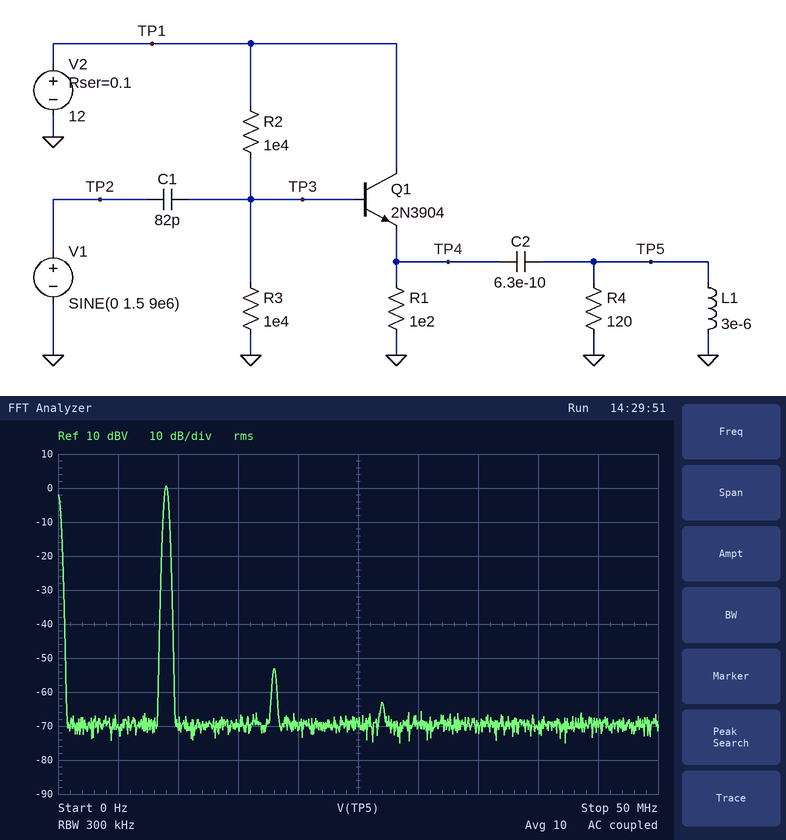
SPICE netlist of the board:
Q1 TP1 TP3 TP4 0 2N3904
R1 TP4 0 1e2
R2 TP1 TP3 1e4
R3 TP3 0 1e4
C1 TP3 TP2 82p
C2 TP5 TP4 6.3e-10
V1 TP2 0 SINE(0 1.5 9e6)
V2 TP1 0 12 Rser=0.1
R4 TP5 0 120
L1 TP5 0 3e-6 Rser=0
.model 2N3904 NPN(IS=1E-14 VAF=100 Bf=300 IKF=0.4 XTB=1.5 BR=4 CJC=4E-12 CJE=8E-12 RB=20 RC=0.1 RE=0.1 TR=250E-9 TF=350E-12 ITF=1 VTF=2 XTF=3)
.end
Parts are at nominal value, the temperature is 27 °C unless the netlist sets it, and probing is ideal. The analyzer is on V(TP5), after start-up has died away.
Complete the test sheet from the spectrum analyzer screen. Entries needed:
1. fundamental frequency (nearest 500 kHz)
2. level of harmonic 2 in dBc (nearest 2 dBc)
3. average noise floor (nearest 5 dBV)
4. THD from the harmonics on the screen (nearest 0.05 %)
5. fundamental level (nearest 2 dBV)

9.0 MHz
-54 dBc
-70 dBV
0.20 %
0 dBV
